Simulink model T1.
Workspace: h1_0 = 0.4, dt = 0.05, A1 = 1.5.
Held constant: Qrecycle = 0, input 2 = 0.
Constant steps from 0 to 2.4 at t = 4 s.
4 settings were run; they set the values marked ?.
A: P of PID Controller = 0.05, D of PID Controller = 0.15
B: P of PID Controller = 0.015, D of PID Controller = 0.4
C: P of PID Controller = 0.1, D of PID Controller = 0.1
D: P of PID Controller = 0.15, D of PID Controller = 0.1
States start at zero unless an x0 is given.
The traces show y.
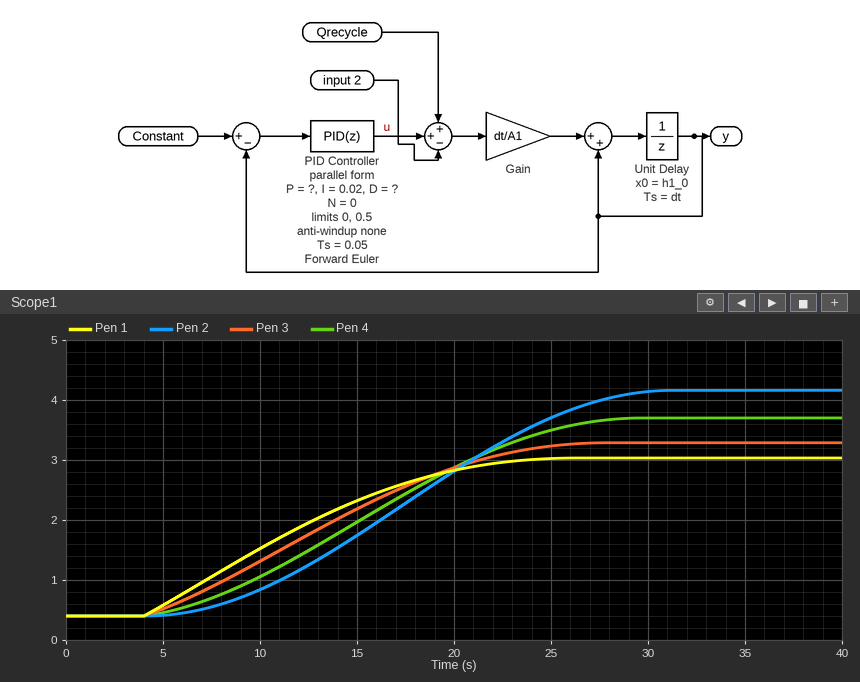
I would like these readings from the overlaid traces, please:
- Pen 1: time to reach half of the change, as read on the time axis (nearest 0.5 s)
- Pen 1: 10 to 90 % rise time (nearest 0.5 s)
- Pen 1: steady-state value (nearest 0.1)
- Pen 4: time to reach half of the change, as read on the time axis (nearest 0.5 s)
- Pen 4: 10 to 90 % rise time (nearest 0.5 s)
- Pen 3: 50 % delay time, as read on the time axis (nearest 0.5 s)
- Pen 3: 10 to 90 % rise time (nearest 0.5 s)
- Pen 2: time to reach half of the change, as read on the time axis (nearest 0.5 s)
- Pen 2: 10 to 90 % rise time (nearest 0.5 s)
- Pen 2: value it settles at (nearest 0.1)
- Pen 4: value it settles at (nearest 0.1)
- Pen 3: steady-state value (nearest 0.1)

11.0 s
14.0 s
3.0
15.5 s
16.0 s
13.0 s
15.0 s
17.5 s
16.0 s
4.2
3.7
3.3
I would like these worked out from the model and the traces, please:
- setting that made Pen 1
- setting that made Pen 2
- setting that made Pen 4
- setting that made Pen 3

D
B
A
C
